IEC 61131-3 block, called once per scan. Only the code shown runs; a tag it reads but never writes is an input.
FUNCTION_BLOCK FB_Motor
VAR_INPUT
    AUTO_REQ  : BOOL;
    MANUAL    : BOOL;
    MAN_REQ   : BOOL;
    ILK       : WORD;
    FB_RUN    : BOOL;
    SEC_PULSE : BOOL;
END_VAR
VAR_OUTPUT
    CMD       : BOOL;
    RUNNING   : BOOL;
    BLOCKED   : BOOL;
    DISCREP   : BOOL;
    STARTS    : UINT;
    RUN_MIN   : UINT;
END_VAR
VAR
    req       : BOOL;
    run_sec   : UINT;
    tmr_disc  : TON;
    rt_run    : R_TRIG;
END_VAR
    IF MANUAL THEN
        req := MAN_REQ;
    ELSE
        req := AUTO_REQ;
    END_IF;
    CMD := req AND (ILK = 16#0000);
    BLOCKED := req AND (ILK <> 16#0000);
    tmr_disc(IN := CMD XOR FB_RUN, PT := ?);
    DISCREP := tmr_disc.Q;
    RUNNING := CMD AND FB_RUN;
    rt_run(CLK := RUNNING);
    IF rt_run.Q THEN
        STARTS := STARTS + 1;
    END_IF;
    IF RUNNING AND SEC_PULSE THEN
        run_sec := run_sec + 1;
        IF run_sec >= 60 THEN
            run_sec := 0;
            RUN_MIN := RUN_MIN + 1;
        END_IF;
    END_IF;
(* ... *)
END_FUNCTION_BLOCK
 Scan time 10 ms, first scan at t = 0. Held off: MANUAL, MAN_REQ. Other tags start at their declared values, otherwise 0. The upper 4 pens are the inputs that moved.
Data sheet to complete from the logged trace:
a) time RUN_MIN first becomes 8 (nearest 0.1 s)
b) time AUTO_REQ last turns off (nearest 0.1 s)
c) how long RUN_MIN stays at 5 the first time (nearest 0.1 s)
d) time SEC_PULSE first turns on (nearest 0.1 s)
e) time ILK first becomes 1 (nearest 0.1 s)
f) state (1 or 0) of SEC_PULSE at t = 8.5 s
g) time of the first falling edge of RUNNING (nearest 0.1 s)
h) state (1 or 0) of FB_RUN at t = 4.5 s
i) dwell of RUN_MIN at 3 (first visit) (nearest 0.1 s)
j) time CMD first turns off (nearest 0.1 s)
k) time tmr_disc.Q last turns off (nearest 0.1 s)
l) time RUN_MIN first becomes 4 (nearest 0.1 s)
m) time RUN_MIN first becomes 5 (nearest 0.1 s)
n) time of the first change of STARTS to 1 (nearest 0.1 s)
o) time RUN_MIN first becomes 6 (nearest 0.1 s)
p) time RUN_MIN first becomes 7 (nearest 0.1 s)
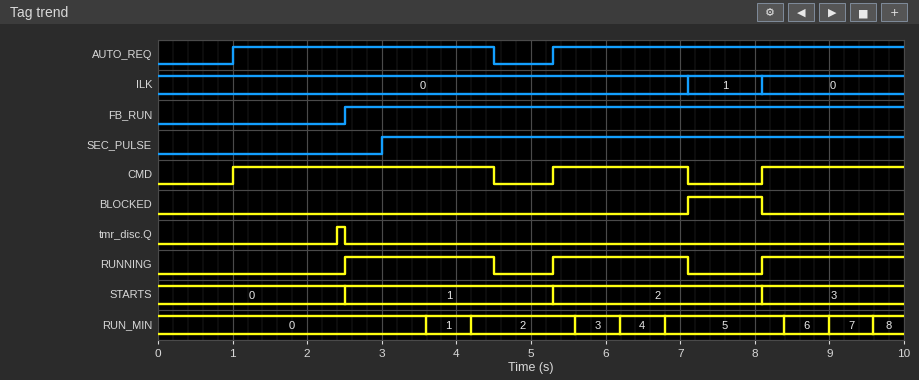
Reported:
9.6 s
4.5 s
1.6 s
3.0 s
7.1 s
1
4.5 s
1
0.6 s
4.5 s
2.5 s
6.2 s
6.8 s
2.5 s
8.4 s
9.0 s
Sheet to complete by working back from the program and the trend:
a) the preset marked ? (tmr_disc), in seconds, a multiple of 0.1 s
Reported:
1.4 s
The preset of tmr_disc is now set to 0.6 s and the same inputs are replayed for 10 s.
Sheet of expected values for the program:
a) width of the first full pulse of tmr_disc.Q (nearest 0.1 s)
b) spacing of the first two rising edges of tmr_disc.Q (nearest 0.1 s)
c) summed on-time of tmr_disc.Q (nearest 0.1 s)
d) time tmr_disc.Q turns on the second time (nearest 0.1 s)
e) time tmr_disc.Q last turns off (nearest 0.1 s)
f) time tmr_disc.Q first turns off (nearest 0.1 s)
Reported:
0.9 s
3.5 s
1.5 s
5.1 s
8.1 s
2.5 s
